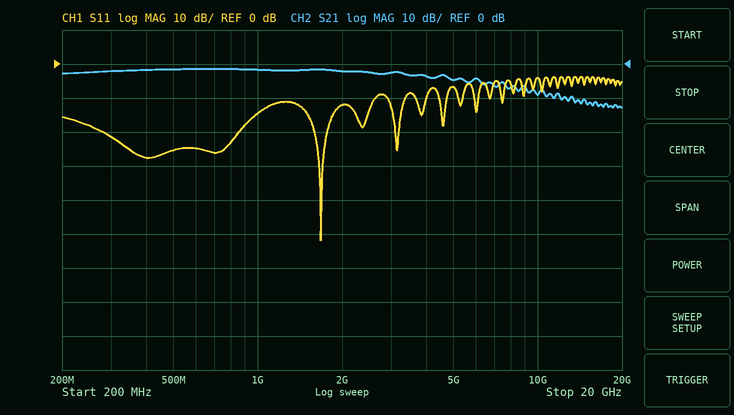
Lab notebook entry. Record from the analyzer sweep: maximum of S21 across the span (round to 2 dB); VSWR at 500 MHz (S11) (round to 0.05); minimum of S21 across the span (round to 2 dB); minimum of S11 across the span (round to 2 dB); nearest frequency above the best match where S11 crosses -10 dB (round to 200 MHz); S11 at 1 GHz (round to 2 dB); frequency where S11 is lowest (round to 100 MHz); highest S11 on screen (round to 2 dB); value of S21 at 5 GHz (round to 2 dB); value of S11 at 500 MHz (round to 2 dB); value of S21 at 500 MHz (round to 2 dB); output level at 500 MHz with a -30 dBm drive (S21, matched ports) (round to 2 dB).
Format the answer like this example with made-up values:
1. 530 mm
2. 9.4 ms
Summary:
1. -2 dB
2. 1.10
3. -12 dB
4. -52 dB
5. 2.6 GHz
6. -14 dB
7. 1.7 GHz
8. -4 dB
9. -4 dB
10. -26 dB
11. -2 dB
12. -32 dBm
